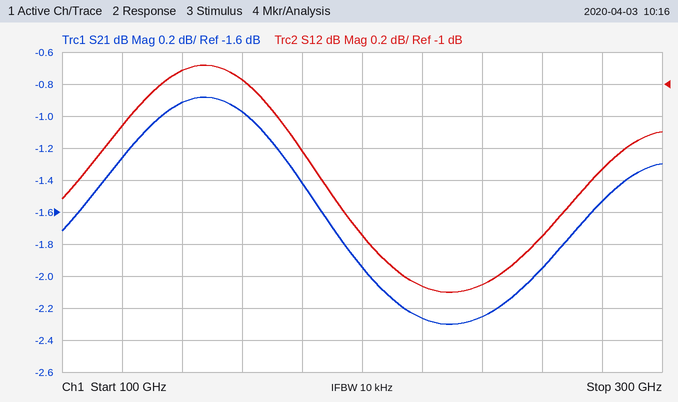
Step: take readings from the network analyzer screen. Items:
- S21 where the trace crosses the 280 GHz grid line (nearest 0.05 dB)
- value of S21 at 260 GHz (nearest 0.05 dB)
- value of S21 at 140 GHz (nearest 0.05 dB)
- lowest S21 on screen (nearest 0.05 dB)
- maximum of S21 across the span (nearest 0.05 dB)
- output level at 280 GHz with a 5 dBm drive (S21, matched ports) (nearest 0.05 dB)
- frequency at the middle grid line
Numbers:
-1.55 dB
-1.95 dB
-0.90 dB
-2.30 dB
-0.90 dB
3.45 dBm
200 GHz
